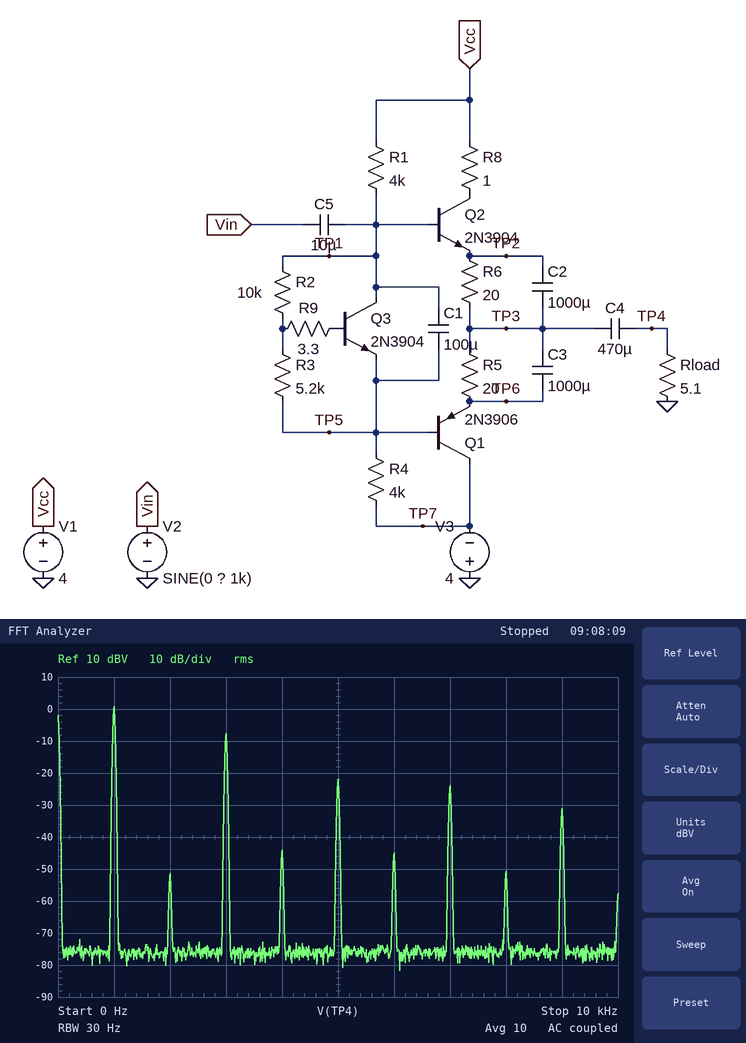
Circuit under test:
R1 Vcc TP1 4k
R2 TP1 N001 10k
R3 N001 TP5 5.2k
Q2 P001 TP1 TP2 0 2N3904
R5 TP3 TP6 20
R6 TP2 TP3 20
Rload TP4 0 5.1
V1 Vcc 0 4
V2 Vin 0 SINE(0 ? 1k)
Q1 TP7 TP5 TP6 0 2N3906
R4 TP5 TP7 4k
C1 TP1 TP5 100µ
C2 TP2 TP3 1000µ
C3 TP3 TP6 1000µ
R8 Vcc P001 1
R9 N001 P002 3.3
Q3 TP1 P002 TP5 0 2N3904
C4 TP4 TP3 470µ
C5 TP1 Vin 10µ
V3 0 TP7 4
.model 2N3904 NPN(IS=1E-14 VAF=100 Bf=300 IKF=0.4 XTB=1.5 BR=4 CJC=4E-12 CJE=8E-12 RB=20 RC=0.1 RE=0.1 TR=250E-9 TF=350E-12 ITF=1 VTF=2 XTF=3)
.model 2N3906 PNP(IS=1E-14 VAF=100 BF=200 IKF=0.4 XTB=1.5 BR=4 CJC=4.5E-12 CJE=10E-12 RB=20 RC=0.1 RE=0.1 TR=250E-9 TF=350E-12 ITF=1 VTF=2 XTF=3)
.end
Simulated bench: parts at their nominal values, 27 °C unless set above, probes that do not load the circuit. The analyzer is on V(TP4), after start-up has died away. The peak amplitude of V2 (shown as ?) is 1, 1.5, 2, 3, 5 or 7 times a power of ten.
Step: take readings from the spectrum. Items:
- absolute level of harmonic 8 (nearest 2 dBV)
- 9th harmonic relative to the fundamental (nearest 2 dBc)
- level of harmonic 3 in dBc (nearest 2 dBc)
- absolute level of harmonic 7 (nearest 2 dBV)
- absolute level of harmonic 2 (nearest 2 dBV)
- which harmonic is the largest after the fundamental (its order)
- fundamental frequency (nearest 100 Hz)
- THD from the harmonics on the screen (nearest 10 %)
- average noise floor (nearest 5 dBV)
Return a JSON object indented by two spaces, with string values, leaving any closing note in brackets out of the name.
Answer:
{
  "absolute level of harmonic 8": "-50 dBV",
  "9th harmonic relative to the fundamental": "-32 dBc",
  "level of harmonic 3 in dBc": "-8 dBc",
  "absolute level of harmonic 7": "-24 dBV",
  "absolute level of harmonic 2": "-52 dBV",
  "which harmonic is the largest after the fundamental": "3",
  "fundamental frequency": "1.0 kHz",
  "THD from the harmonics on the screen": "40 %",
  "average noise floor": "-75 dBV"
}
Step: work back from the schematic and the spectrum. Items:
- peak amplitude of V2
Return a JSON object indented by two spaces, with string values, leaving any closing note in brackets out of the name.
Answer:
{
  "peak amplitude of V2": "5 V"
}
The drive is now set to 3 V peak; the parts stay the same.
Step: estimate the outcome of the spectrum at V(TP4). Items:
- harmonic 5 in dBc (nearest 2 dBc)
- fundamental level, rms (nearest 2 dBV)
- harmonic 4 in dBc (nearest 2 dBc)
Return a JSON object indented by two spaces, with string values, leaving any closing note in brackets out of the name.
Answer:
{
  "harmonic 5 in dBc": "-22 dBc",
  "fundamental level, rms": "0 dBV",
  "harmonic 4 in dBc": "-56 dBc"
}
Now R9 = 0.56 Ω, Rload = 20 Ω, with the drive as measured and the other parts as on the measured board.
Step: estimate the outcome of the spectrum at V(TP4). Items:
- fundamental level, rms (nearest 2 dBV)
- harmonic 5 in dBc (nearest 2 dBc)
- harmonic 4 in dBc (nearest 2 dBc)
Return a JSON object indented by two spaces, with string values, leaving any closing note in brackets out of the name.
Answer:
{
  "fundamental level, rms": "6 dBV",
  "harmonic 5 in dBc": "-20 dBc",
  "harmonic 4 in dBc": "-58 dBc"
}
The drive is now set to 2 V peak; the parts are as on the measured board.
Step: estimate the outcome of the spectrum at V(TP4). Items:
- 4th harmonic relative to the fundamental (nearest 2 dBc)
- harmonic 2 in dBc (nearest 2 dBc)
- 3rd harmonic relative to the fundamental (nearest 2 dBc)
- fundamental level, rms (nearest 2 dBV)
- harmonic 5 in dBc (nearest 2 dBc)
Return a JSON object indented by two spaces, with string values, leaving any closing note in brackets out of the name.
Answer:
{
  "4th harmonic relative to the fundamental": "-58 dBc",
  "harmonic 2 in dBc": "-54 dBc",
  "3rd harmonic relative to the fundamental": "-12 dBc",
  "fundamental level, rms": "-4 dBV",
  "harmonic 5 in dBc": "-22 dBc"
}
